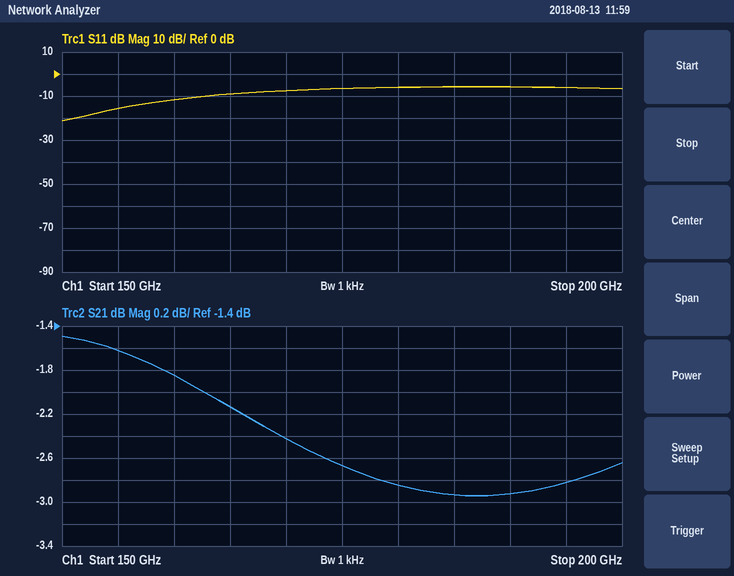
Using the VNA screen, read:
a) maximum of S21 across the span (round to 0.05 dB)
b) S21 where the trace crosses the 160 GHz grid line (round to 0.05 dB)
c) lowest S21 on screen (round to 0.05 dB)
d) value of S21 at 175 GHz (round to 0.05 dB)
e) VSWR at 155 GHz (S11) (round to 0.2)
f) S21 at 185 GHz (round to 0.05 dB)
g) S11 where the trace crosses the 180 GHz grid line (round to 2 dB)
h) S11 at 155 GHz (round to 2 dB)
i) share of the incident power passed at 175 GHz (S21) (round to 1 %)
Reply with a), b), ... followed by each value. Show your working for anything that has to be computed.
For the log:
a) -1.50 dB
b) -1.85 dB
c) -2.95 dB
d) -2.65 dB
e) |Γ| = 10^(-16/20) = 0.1585; VSWR = (1 + 0.1585)/(1 − 0.1585) ≈ 1.4
f) -2.95 dB
g) -6 dB
h) -16 dB
i) 10^(-2.65/10) ≈ 54 %
